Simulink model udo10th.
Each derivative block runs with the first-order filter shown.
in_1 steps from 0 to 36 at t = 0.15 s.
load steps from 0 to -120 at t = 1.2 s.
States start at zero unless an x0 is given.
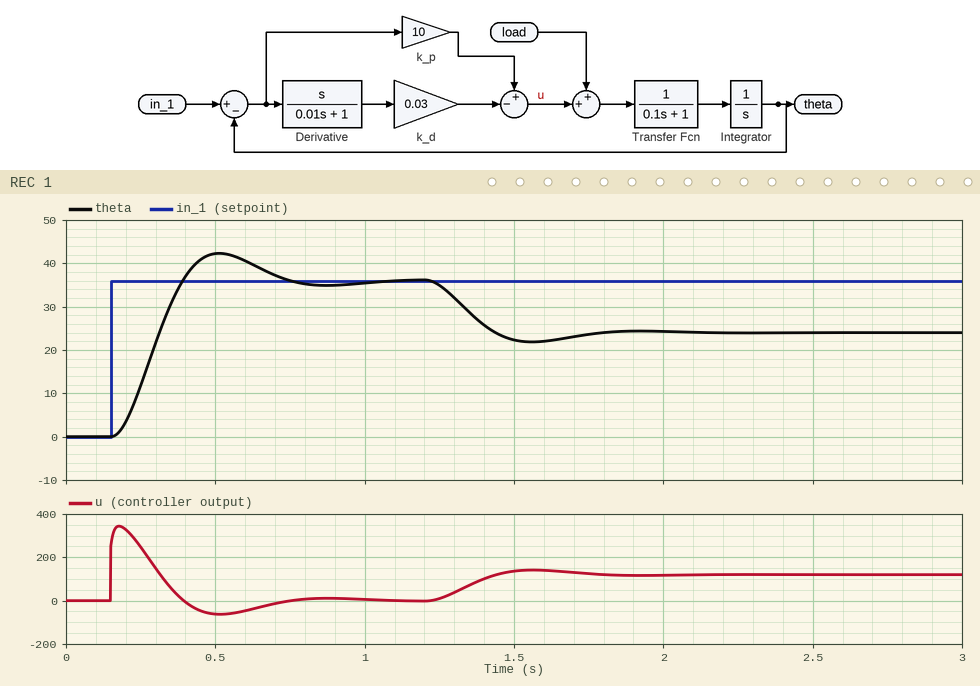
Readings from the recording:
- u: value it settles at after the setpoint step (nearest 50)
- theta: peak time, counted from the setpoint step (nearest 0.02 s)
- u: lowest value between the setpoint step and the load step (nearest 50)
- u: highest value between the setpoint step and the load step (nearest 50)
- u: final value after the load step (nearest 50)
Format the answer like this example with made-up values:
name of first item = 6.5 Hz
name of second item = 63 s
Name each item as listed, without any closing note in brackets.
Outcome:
u: value it settles at after the setpoint step = 0
theta: peak time, counted from the setpoint step = 0.36 s
u: lowest value between the setpoint step and the load step = -50
u: highest value between the setpoint step and the load step = 350
u: final value after the load step = 100
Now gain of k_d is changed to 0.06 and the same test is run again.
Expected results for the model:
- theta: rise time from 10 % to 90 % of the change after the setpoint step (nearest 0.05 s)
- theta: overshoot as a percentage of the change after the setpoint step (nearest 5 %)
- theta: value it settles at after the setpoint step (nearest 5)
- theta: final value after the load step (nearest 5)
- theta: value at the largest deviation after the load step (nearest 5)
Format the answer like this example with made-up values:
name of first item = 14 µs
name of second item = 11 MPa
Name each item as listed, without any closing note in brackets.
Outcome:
theta: rise time from 10 % to 90 % of the change after the setpoint step = 0.15 s
theta: overshoot as a percentage of the change after the setpoint step = 20 %
theta: value it settles at after the setpoint step = 35
theta: final value after the load step = 25
theta: value at the largest deviation after the load step = 20
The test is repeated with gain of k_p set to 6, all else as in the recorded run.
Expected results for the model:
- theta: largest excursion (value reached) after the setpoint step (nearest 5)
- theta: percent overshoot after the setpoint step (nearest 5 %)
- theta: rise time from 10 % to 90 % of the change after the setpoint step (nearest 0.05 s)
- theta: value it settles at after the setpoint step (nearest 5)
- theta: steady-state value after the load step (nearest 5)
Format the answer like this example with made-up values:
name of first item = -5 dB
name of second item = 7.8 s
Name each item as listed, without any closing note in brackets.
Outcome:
theta: largest excursion (value reached) after the setpoint step = 40
theta: percent overshoot after the setpoint step = 10 %
theta: rise time from 10 % to 90 % of the change after the setpoint step = 0.25 s
theta: value it settles at after the setpoint step = 35
theta: steady-state value after the load step = 15
